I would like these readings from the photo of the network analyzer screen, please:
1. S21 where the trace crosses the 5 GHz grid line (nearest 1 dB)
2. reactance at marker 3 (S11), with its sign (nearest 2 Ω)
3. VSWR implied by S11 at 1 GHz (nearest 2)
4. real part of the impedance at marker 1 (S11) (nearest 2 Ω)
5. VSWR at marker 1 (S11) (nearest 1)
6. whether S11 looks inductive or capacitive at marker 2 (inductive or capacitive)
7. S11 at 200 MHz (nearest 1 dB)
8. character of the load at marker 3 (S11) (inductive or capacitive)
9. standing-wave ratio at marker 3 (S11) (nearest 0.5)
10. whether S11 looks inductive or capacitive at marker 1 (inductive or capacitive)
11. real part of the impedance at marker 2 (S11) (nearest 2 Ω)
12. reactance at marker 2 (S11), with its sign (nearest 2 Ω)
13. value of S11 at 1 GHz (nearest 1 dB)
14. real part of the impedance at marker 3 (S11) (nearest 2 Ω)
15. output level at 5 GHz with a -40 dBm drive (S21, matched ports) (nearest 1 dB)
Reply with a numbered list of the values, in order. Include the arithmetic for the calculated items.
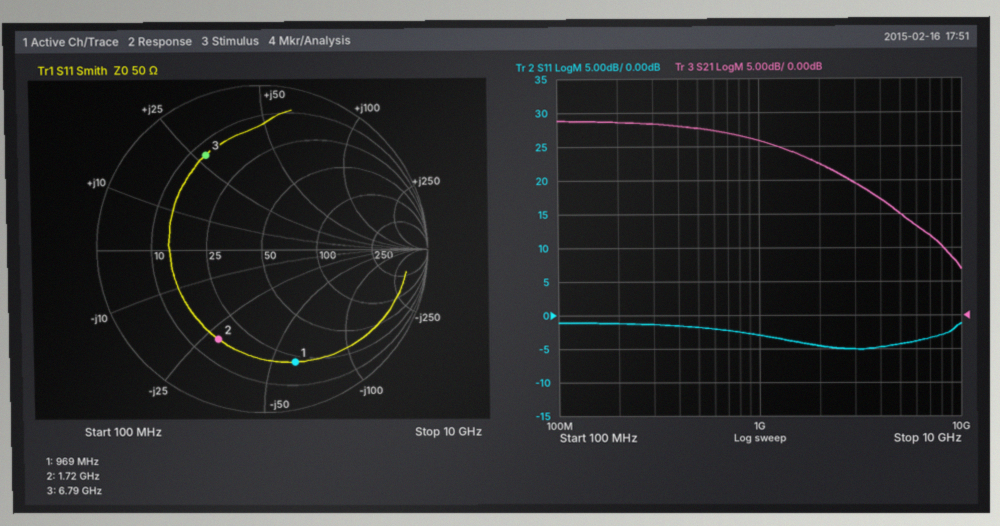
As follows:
1. 15 dB
2. +28 Ω
3. |Γ| = 10^(-3/20) = 0.7079; VSWR = (1 + 0.7079)/(1 − 0.7079) ≈ 6
4. 22 Ω
5. 6
6. capacitive
7. -1 dB
8. inductive
9. 5.0
10. capacitive
11. 16 Ω
12. -28 Ω
13. -3 dB
14. 14 Ω
15. -40 dBm + (15 dB) = -25 dBm
